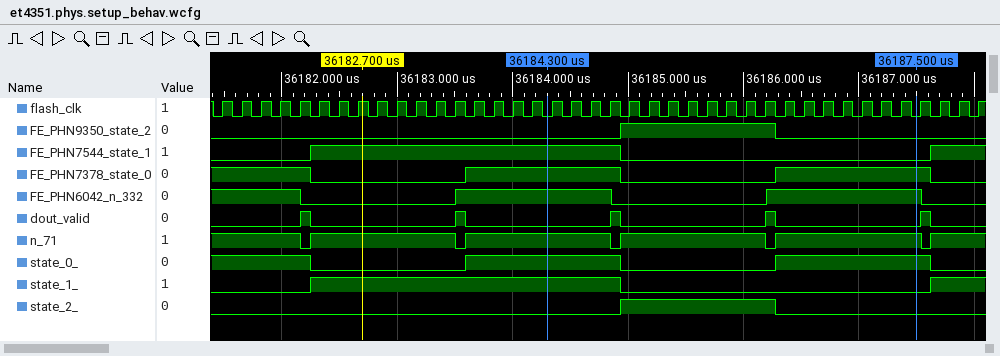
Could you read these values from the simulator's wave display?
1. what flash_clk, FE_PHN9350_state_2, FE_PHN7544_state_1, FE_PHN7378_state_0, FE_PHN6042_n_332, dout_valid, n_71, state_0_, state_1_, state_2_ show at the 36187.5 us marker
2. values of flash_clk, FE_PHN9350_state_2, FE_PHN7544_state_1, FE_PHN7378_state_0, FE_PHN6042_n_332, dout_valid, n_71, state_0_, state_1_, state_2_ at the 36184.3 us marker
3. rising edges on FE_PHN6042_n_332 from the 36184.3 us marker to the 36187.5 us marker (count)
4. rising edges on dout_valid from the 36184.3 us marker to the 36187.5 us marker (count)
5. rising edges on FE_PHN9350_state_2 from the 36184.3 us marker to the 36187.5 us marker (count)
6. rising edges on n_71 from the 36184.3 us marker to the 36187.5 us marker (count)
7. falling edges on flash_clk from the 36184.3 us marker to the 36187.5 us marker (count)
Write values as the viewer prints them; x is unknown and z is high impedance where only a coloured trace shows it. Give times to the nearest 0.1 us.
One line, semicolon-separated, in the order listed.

flash_clk=0, FE_PHN9350_state_2=0, FE_PHN7544_state_1=0, FE_PHN7378_state_0=1, FE_PHN6042_n_332=1, dout_valid=0, n_71=1, state_0_=1, state_1_=0, state_2_=0; flash_clk=0, FE_PHN9350_state_2=0, FE_PHN7544_state_1=1, FE_PHN7378_state_0=1, FE_PHN6042_n_332=1, dout_valid=0, n_71=1, state_0_=1, state_1_=1, state_2_=0; 1; 2; 1; 2; 19
